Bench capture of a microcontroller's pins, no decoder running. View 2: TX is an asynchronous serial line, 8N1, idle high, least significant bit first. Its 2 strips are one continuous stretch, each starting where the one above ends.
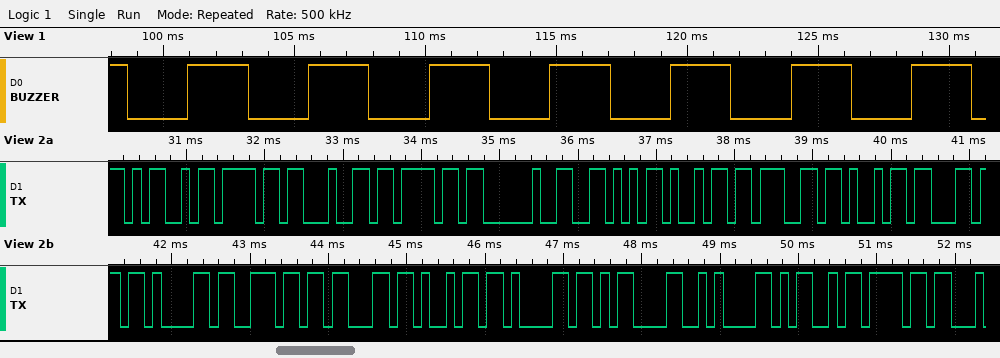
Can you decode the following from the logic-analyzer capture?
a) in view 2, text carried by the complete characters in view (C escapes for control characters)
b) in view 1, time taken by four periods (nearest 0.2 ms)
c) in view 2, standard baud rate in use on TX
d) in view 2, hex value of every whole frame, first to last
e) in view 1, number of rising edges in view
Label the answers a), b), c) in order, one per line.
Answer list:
a) "Modo Vigilancia\r\nMo"
b) 18.4 ms
c) 9600 baud
d) 4D 6F 64 6F 20 56 69 67 69 6C 61 6E 63 69 61 0D 0A 4D 6F
e) 7
